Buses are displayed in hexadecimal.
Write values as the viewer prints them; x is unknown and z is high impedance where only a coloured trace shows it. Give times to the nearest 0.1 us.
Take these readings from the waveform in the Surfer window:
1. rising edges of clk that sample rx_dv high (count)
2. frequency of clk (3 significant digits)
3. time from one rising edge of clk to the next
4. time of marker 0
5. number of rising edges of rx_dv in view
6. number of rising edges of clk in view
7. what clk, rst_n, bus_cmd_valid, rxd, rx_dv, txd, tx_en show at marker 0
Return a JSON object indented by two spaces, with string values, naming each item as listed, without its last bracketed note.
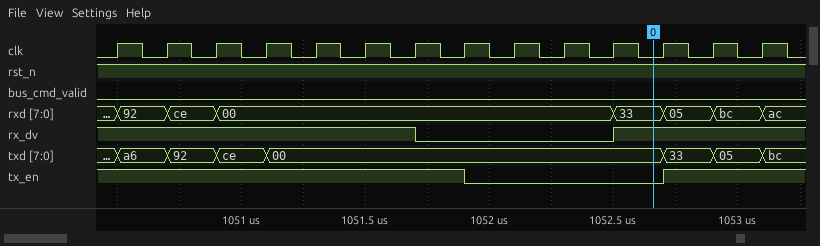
{
  "rising edges of clk that sample rx_dv high": "10",
  "frequency of clk": "5.00 MHz",
  "time from one rising edge of clk to the next": "0.2 us",
  "time of marker 0": "1052.7 us",
  "number of rising edges of rx_dv in view": "1",
  "number of rising edges of clk in view": "14",
  "what clk, rst_n, bus_cmd_valid, rxd, rx_dv, txd, tx_en show at marker 0": "clk=0, rst_n=1, bus_cmd_valid=0, rxd=33, rx_dv=1, txd=00, tx_en=0"
}
